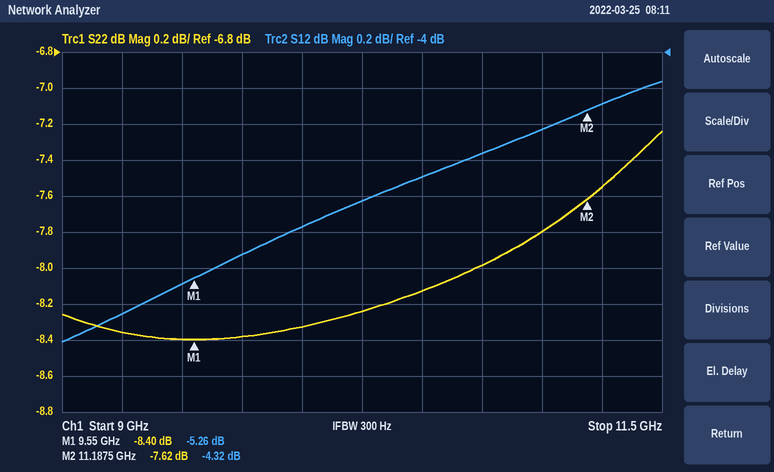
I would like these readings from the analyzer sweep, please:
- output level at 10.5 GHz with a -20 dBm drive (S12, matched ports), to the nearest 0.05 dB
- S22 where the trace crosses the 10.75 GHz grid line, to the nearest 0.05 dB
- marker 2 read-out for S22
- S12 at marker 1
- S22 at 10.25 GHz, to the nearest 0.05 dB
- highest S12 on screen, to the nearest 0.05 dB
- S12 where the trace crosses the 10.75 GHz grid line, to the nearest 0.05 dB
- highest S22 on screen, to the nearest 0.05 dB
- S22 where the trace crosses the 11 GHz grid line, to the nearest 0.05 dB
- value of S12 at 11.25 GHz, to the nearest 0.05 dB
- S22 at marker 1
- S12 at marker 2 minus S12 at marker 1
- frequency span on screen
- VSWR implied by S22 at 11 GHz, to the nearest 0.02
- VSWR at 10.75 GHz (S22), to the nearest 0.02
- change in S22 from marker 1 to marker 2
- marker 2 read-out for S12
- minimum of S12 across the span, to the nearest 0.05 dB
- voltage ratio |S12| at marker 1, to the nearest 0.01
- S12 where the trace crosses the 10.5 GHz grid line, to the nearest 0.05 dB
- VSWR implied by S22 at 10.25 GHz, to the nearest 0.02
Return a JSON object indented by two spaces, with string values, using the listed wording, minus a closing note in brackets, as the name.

{
  "output level at 10.5 GHz with a -20 dBm drive (S12, matched ports), to the nearest 0.05 dB": "-24.70 dBm",
  "S22 where the trace crosses the 10.75 GHz grid line, to the nearest 0.05 dB": "-8.00 dB",
  "marker 2 read-out for S22": "-7.62 dB",
  "S12 at marker 1": "-5.26 dB",
  "S22 at 10.25 GHz, to the nearest 0.05 dB": "-8.25 dB",
  "highest S12 on screen, to the nearest 0.05 dB": "-4.15 dB",
  "S12 where the trace crosses the 10.75 GHz grid line, to the nearest 0.05 dB": "-4.55 dB",
  "highest S22 on screen, to the nearest 0.05 dB": "-7.25 dB",
  "S22 where the trace crosses the 11 GHz grid line, to the nearest 0.05 dB": "-7.80 dB",
  "value of S12 at 11.25 GHz, to the nearest 0.05 dB": "-4.30 dB",
  "S22 at marker 1": "-8.40 dB",
  "S12 at marker 2 minus S12 at marker 1": "0.94 dB",
  "frequency span on screen": "2.5 GHz",
  "VSWR implied by S22 at 11 GHz, to the nearest 0.02": "2.38",
  "VSWR at 10.75 GHz (S22), to the nearest 0.02": "2.32",
  "change in S22 from marker 1 to marker 2": "0.78 dB",
  "marker 2 read-out for S12": "-4.32 dB",
  "minimum of S12 across the span, to the nearest 0.05 dB": "-5.60 dB",
  "voltage ratio |S12| at marker 1, to the nearest 0.01": "0.55",
  "S12 where the trace crosses the 10.5 GHz grid line, to the nearest 0.05 dB": "-4.70 dB",
  "VSWR implied by S22 at 10.25 GHz, to the nearest 0.02": "2.26"
}
